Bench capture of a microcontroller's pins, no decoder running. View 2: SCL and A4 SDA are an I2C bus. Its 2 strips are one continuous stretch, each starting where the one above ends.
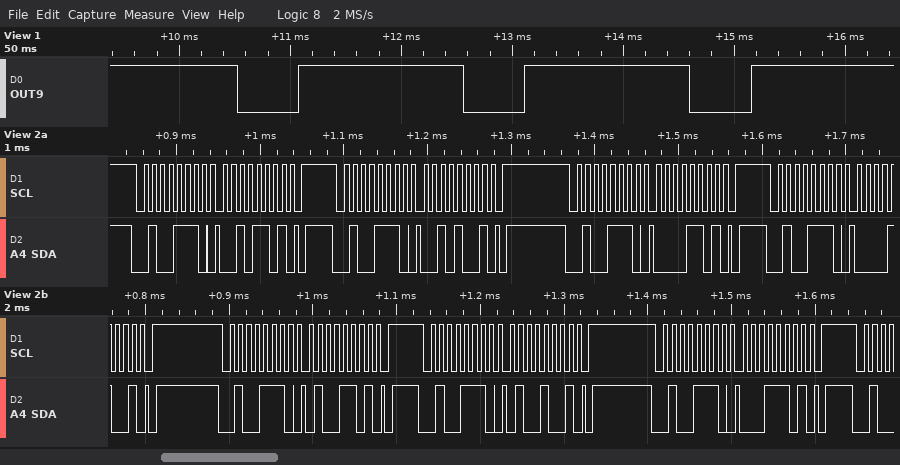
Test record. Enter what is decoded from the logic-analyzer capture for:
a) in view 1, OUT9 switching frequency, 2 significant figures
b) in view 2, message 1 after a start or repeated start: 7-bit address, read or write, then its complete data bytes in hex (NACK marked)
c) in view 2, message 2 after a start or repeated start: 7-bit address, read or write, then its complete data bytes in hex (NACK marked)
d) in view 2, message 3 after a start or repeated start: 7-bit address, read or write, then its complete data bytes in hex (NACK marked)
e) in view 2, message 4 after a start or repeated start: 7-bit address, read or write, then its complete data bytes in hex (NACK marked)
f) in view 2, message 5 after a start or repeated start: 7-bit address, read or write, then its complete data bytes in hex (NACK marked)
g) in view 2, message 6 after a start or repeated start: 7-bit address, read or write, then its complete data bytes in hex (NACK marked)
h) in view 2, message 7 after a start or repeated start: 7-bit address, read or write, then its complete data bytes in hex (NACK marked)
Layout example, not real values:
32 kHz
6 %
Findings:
490 Hz
0x27 write: 2D
0x27 write: 29
0x27 write: 0D
0x27 write: 09
0x27 write: 4D
0x27 write: 49
0x27 write: 1D
